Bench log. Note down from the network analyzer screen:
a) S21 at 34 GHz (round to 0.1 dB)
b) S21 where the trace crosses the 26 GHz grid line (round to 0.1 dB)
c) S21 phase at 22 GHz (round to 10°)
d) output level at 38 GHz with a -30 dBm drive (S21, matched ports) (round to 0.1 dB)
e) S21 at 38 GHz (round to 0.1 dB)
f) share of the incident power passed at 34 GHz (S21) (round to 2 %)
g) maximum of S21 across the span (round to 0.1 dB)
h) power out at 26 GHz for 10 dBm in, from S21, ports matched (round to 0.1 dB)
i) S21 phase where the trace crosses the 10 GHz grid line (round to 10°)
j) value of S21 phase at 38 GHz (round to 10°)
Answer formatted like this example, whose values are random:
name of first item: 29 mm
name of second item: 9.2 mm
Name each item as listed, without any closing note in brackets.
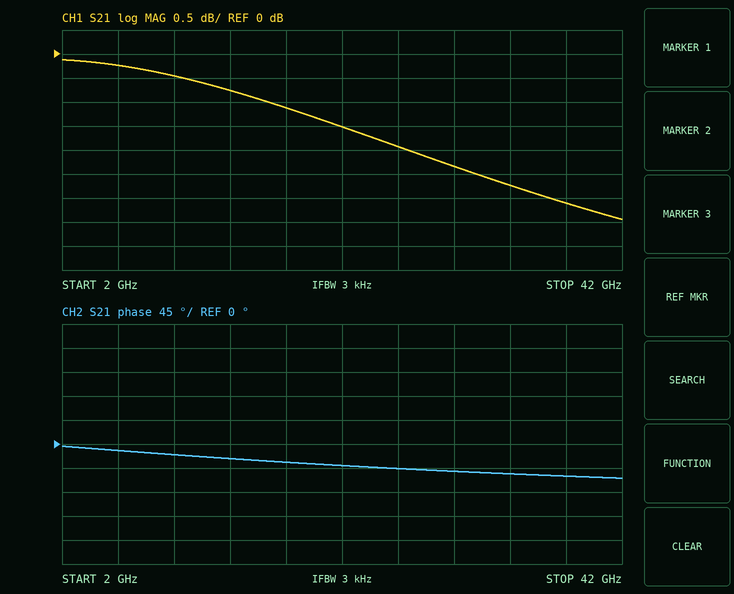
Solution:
S21 at 34 GHz: -2.7 dB
S21 where the trace crosses the 26 GHz grid line: -1.9 dB
S21 phase at 22 GHz: -40°
output level at 38 GHz with a -30 dBm drive (S21, matched ports): -33.1 dBm
S21 at 38 GHz: -3.1 dB
share of the incident power passed at 34 GHz (S21): 54 %
maximum of S21 across the span: -0.1 dB
power out at 26 GHz for 10 dBm in, from S21, ports matched: 8.1 dBm
S21 phase where the trace crosses the 10 GHz grid line: -20°
value of S21 phase at 38 GHz: -60°
